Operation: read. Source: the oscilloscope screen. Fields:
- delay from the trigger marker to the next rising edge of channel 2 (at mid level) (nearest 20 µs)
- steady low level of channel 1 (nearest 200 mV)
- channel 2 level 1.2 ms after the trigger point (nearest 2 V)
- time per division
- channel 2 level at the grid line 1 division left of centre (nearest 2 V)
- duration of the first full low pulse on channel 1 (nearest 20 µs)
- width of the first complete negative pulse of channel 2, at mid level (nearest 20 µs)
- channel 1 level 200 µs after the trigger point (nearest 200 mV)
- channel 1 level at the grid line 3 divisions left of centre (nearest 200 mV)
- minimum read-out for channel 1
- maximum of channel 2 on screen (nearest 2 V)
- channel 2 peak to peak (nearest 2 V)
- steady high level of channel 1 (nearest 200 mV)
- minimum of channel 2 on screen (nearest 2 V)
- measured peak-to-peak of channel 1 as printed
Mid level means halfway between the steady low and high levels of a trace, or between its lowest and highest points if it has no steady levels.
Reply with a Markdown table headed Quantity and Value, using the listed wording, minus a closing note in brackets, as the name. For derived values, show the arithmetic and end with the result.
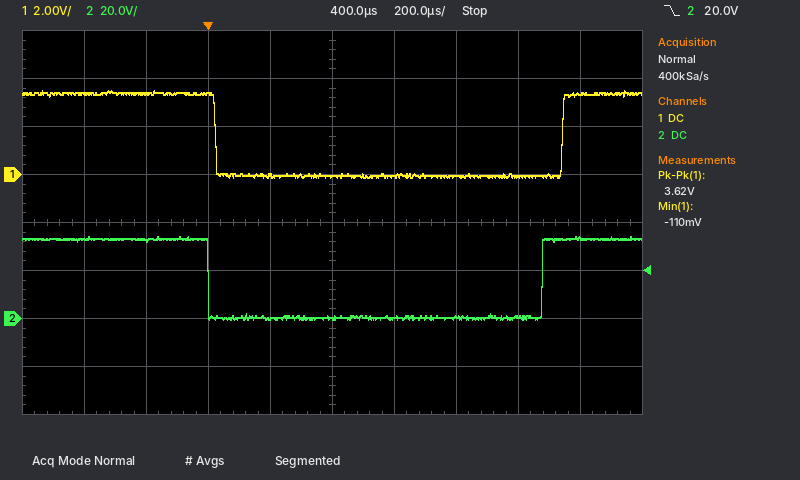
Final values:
| Quantity | Value |
|---|---|
| delay from the trigger marker to the next rising edge of channel 2 (at mid level) | 1.08 ms |
| steady low level of channel 1 | 0.0 V |
| channel 2 level 1.2 ms after the trigger point | 34 V |
| time per division | 200 µs |
| channel 2 level at the grid line 1 division left of centre | 0 V |
| duration of the first full low pulse on channel 1 | 1.12 ms |
| width of the first complete negative pulse of channel 2, at mid level | 1.08 ms |
| channel 1 level 200 µs after the trigger point | 0.0 V |
| channel 1 level at the grid line 3 divisions left of centre | 3.4 V |
| minimum read-out for channel 1 | -110 mV |
| maximum of channel 2 on screen | 34 V |
| channel 2 peak to peak | 34 V − (0 V) = 34 V |
| steady high level of channel 1 | 3.4 V |
| minimum of channel 2 on screen | 0 V |
| measured peak-to-peak of channel 1 as printed | 3.62 V |
